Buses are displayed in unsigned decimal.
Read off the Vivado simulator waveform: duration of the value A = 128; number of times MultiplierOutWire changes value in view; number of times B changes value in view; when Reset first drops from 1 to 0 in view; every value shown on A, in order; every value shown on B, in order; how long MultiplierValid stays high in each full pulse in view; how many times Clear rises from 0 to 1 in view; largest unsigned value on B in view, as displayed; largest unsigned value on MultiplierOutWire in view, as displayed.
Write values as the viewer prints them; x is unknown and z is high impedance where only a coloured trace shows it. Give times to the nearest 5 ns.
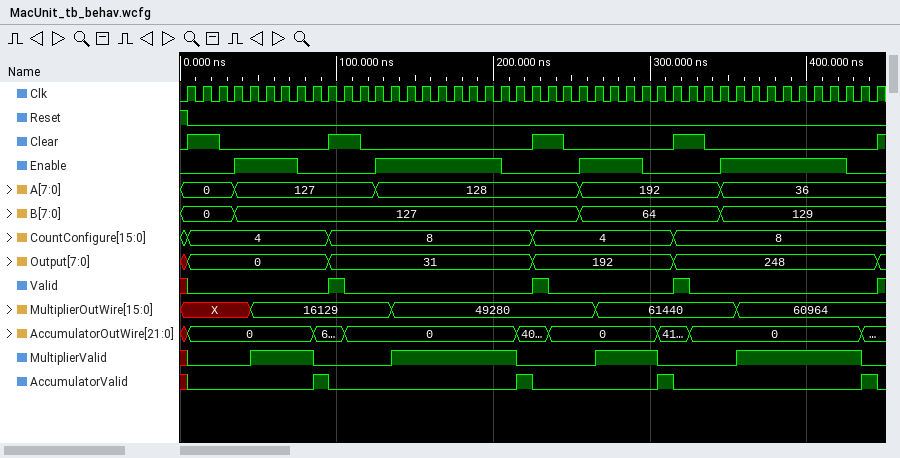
130 ns
4
3
5 ns
0, 127, 128, 192, 36
0, 127, 64, 129
40 ns, 80 ns, 40 ns, 80 ns
5
129
61440
